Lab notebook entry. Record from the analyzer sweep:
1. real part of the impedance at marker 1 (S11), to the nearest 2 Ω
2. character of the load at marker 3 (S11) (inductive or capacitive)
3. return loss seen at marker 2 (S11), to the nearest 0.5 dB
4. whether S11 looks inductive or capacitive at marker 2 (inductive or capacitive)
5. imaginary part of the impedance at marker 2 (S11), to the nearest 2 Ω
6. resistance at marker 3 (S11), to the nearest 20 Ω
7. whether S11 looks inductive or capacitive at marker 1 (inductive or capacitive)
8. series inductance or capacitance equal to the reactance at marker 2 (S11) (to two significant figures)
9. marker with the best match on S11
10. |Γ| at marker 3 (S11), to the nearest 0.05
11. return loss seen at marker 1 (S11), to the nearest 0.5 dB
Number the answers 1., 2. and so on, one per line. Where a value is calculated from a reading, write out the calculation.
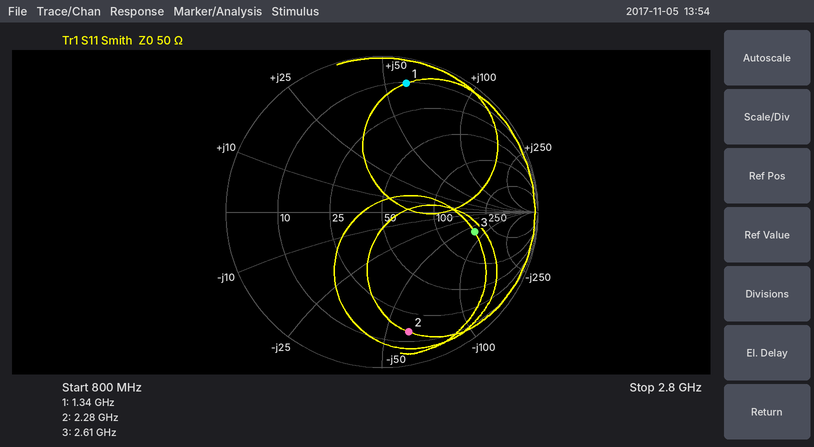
1. 10 Ω
2. capacitive
3. 2.0 dB
4. capacitive
5. -60 Ω
6. 180 Ω
7. inductive
8. C = 1/(2π × 2.28 GHz × 60 Ω) ≈ 1.2 pF
9. marker 3
10. 0.60
11. 1.5 dB
